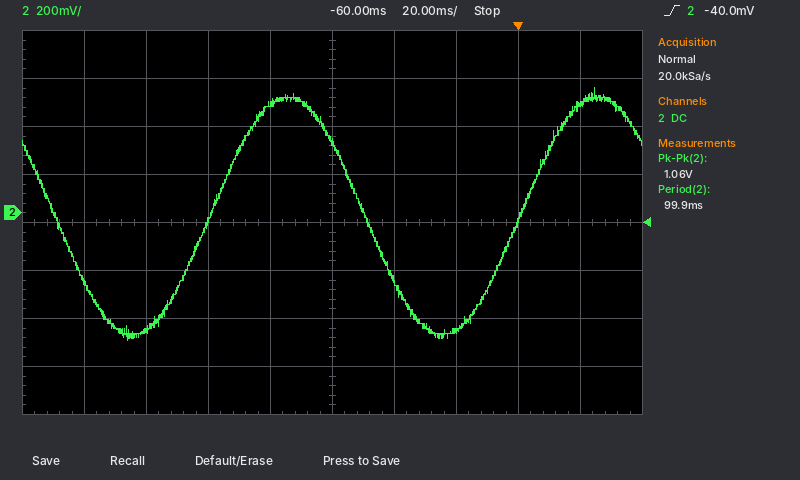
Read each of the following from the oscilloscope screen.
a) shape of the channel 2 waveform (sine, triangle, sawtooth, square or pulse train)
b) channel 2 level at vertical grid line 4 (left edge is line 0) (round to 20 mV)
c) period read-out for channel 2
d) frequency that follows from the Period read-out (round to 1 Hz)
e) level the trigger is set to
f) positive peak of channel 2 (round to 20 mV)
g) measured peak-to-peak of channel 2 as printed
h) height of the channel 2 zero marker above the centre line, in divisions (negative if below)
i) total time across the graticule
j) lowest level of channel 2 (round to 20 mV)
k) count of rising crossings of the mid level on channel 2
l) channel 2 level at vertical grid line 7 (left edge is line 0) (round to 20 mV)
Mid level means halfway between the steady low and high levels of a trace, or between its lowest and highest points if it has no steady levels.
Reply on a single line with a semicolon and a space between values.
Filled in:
sine; 460 mV; 99.9 ms; 10 Hz; -40.0 mV; 520 mV; 1.06 V; +0.2 div; 200 ms; -540 mV; 2; -500 mV
